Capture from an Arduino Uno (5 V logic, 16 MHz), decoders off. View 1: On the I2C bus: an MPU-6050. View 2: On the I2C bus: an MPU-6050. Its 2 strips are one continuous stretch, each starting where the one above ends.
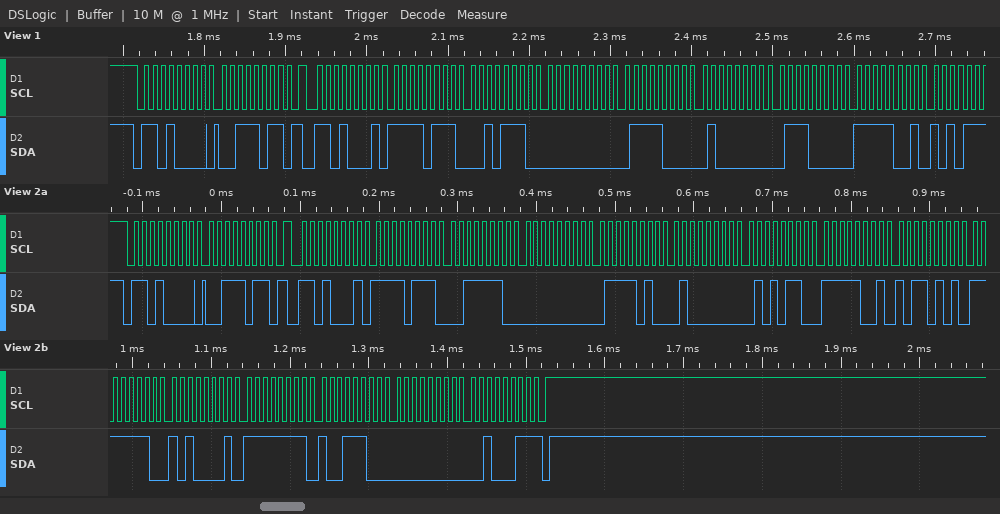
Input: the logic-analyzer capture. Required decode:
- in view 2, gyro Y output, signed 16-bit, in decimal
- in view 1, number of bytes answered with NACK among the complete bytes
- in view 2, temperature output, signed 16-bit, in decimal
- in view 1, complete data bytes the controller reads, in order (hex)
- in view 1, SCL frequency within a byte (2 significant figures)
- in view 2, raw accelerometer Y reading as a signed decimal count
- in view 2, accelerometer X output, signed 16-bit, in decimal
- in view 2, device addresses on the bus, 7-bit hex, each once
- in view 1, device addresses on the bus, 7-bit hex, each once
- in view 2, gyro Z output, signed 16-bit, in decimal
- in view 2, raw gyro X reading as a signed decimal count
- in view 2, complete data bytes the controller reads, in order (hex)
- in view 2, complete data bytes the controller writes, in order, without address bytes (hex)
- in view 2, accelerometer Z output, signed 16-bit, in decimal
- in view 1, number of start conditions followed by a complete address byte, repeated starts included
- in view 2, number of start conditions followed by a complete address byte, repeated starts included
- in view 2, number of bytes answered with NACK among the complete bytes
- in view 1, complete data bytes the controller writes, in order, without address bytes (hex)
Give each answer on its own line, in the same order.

-100
0
-1611
F7 2E 00 78 40 70 F9
100 kHz
122
-2242
0x68
0x68
35
-351
F7 3E 00 7A 40 56 F9 B5 FE A1 FF 9C 00 23
3B
16470
2
2
1
3B
